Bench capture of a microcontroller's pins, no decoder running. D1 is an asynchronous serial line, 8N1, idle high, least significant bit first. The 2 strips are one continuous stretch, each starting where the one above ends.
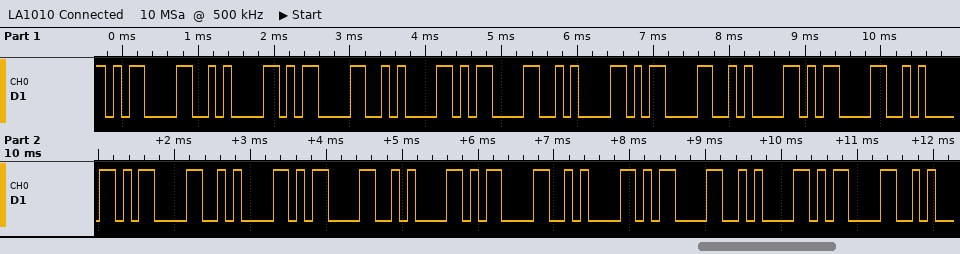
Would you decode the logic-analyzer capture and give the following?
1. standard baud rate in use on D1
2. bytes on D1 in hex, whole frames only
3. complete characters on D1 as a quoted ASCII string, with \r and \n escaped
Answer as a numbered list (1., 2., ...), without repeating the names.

1. 9600 baud
2. 0x0D 0x0A 0x0D 0x0A 0x0D 0x0A 0x0D 0x0A 0x0D 0x0A 0x0D 0x0A 0x0D 0x0A 0x0D 0x0A 0x0D 0x0A 0x0D
3. "\r\n\r\n\r\n\r\n\r\n\r\n\r\n\r\n\r\n\r"
